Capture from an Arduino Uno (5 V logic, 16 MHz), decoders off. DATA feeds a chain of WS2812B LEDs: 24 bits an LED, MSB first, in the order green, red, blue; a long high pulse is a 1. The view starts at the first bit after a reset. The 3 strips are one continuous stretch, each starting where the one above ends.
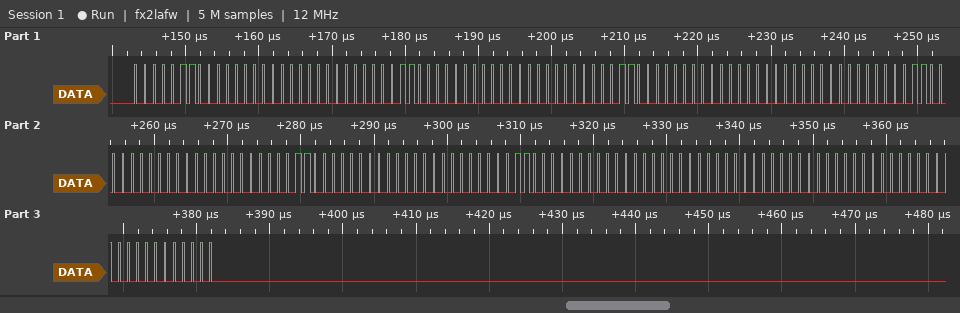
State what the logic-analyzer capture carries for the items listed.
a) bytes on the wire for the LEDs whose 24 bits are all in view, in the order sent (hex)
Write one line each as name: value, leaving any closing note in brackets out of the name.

bytes on the wire for the LEDs whose 24 bits are all in view, in the order sent: 06 00 00 06 00 00 06 00 00 00 06 00 00 06 00 00 06 00 00 00 00 00 00 00
